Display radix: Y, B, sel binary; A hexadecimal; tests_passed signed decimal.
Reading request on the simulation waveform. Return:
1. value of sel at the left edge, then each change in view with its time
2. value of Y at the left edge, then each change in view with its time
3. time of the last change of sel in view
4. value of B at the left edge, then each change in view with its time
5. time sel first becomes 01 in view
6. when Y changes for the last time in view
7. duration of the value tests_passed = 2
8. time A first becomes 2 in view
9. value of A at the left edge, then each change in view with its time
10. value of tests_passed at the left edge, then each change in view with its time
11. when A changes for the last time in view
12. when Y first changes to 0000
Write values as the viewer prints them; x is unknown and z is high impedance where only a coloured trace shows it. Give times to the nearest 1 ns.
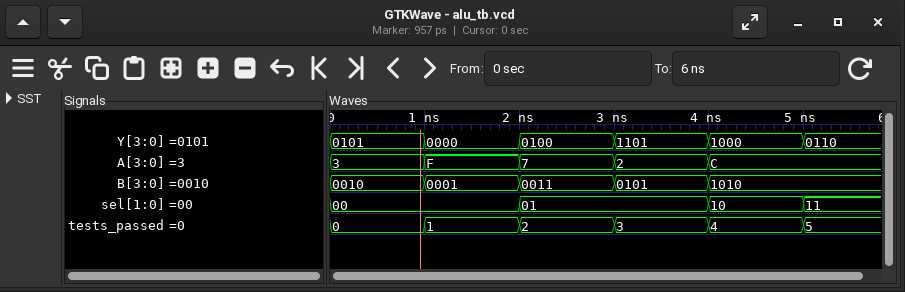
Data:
00, 01 at 2 ns, 10 at 4 ns, 11 at 5 ns
0101, 0000 at 1 ns, 0100 at 2 ns, 1101 at 3 ns, 1000 at 4 ns, 0110 at 5 ns
5 ns
0010, 0001 at 1 ns, 0011 at 2 ns, 0101 at 3 ns, 1010 at 4 ns
2 ns
5 ns
1 ns
3 ns
3, F at 1 ns, 7 at 2 ns, 2 at 3 ns, C at 4 ns
0, 1 at 1 ns, 2 at 2 ns, 3 at 3 ns, 4 at 4 ns, 5 at 5 ns
4 ns
1 ns
